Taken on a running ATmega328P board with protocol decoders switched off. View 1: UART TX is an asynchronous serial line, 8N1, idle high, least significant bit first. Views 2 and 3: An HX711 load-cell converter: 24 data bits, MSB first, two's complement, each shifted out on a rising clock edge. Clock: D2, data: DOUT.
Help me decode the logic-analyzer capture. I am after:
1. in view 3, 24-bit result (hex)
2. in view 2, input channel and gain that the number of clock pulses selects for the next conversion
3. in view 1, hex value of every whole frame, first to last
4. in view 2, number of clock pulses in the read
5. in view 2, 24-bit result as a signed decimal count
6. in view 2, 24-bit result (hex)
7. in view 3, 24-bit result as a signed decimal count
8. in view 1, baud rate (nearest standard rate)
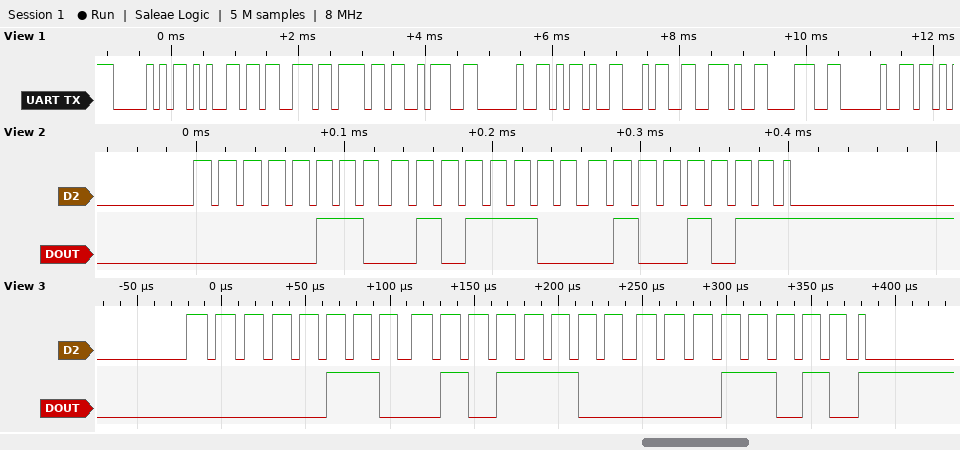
0x065C1A
channel A, gain 128
50 65 73 6F 3A 20 2D 34 2E 38 20
25
416843
0x065C4B
416794
9600 baud
